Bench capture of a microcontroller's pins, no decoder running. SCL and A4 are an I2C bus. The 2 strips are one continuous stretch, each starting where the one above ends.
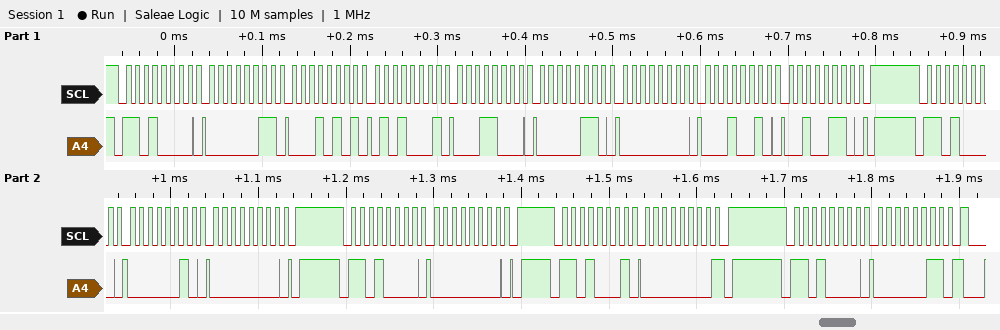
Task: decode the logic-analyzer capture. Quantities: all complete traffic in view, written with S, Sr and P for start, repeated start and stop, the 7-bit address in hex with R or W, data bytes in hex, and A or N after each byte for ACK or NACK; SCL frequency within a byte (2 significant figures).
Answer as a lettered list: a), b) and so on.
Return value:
a) S 68W A 03 A 15 A 51 A 18 A 06 A 00 A 12 A 26 A P S 68W A 02 A 00 A P S 68W A 00 A P S 68R A 00 N P S 68W A 03 A
b) 100 kHz
